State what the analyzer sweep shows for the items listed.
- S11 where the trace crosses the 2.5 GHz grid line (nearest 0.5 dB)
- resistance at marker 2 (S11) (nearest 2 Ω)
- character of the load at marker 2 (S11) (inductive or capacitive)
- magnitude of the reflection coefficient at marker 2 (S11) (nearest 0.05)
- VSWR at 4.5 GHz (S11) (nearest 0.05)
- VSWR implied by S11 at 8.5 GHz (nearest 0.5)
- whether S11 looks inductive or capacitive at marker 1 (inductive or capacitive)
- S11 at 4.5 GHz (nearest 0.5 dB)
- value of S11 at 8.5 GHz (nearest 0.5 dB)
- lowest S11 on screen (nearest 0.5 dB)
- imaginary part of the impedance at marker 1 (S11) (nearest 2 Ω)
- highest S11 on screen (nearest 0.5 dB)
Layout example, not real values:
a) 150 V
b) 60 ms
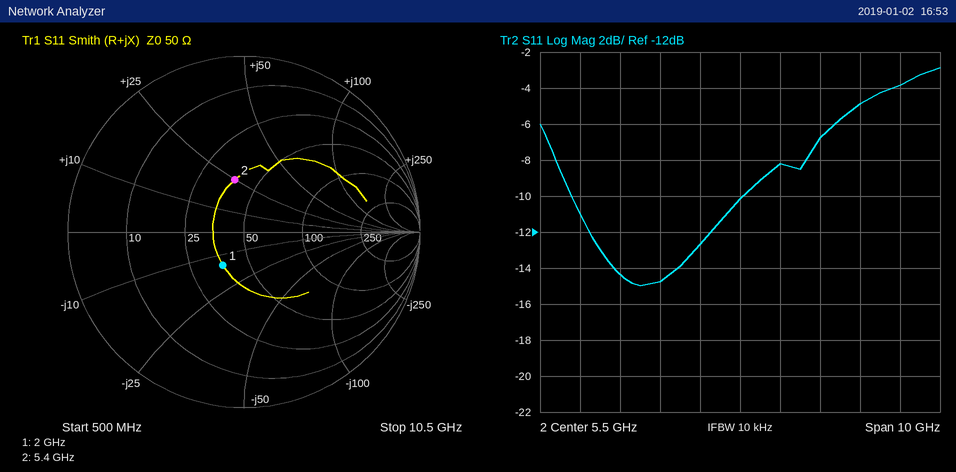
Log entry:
a) -14.5 dB
b) 38 Ω
c) inductive
d) 0.30
e) 1.60
f) 3.5
g) capacitive
h) -12.5 dB
i) -5.0 dB
j) -15.0 dB
k) -14 Ω
l) -3.0 dB
